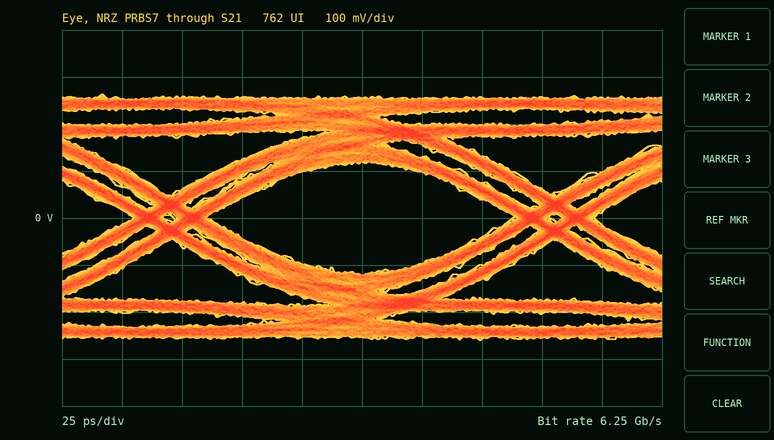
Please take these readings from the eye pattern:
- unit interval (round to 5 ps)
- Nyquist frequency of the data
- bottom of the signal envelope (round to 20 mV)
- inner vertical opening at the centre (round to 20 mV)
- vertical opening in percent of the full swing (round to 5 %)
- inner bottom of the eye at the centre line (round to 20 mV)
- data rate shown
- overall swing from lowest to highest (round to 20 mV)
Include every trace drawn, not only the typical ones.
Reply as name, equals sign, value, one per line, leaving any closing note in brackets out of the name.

unit interval = 160 ps
Nyquist frequency of the data = 3.125 GHz
bottom of the signal envelope = -260 mV
inner vertical opening at the centre = 240 mV
vertical opening in percent of the full swing = 45 %
inner bottom of the eye at the centre line = -120 mV
data rate shown = 6.25 Gb/s
overall swing from lowest to highest = 520 mV
